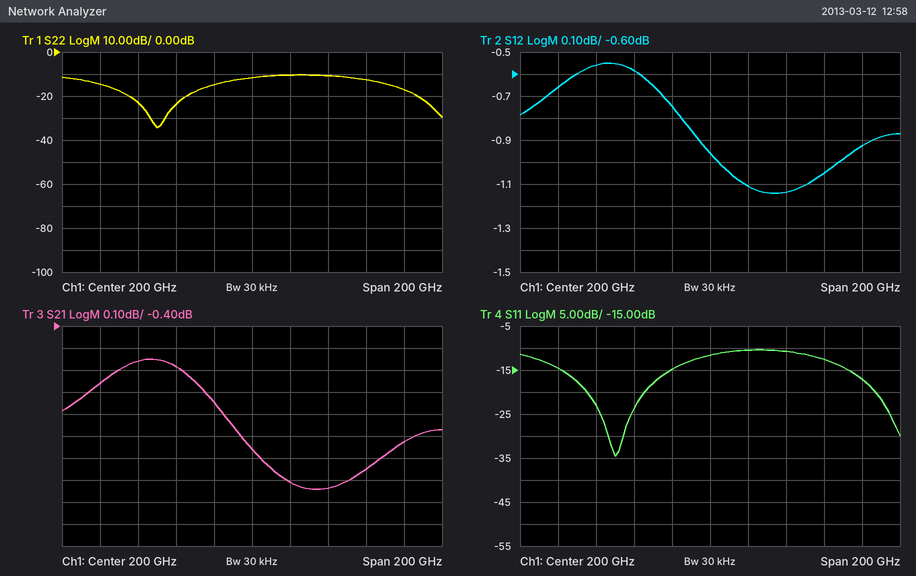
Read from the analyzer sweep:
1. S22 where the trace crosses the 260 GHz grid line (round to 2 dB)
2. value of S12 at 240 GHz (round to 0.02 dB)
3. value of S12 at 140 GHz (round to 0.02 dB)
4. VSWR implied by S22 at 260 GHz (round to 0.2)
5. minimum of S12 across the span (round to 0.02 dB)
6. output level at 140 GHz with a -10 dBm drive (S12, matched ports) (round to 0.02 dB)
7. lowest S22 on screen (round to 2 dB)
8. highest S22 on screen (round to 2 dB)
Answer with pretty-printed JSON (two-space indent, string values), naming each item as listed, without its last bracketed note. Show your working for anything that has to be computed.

{
  "S22 where the trace crosses the 260 GHz grid line": "-12 dB",
  "value of S12 at 240 GHz": "-1.14 dB",
  "value of S12 at 140 GHz": "-0.56 dB",
  "VSWR implied by S22 at 260 GHz": "|Γ| = 10^(-12/20) = 0.2512; VSWR = (1 + 0.2512)/(1 − 0.2512) ≈ 1.67, so 1.6 to the nearest 0.2",
  "minimum of S12 across the span": "-1.14 dB",
  "output level at 140 GHz with a -10 dBm drive (S12, matched ports)": "-10 dBm + (-0.56 dB) = -10.56 dBm",
  "lowest S22 on screen": "-34 dB",
  "highest S22 on screen": "-10 dB"
}
